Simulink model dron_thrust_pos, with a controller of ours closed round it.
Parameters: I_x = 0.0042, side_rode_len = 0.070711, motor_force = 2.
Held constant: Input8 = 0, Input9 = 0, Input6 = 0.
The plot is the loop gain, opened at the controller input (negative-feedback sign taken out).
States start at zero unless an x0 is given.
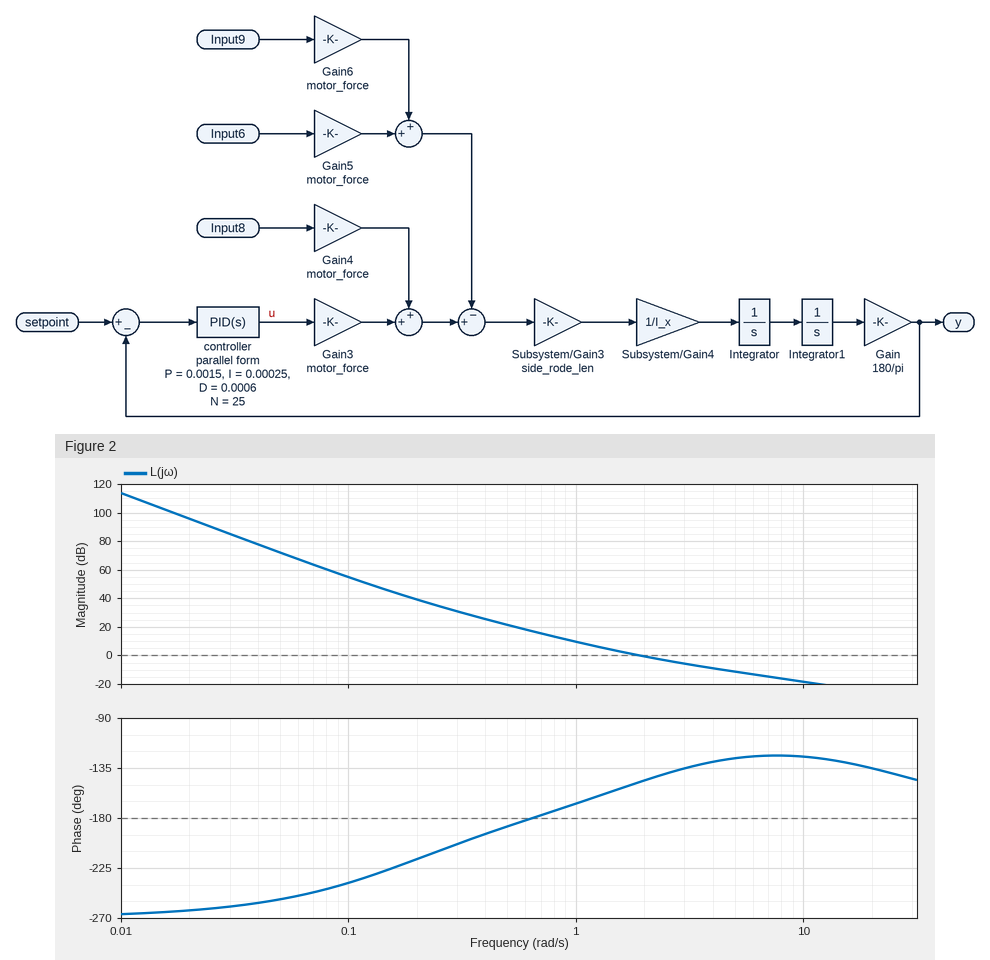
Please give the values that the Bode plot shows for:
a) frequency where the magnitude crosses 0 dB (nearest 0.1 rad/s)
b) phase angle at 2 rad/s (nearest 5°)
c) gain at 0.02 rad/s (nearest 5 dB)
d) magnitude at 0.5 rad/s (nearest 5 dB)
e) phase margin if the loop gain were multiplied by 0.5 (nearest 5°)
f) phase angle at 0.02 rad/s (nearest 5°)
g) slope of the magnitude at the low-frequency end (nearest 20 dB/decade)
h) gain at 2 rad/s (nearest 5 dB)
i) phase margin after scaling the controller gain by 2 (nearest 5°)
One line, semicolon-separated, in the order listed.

1.9 rad/s; -145°; 95 dB; 20 dB; 20°; -265°; -60 dB/decade; 0 dB; 45°
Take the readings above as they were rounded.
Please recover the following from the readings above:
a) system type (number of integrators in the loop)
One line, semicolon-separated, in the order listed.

3
